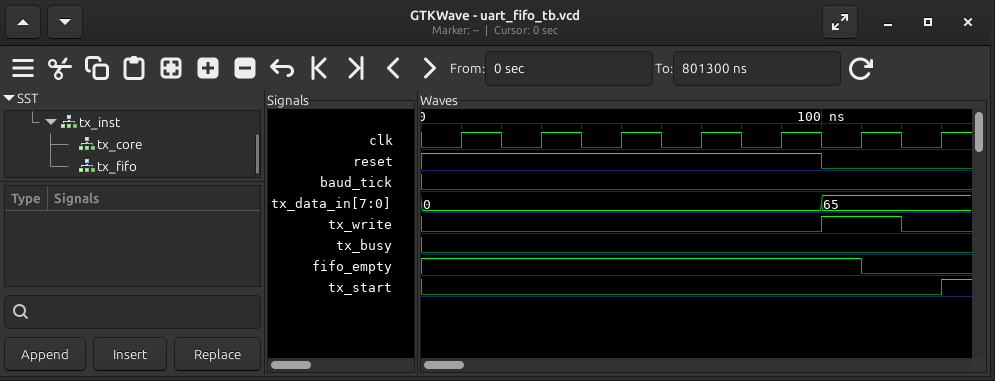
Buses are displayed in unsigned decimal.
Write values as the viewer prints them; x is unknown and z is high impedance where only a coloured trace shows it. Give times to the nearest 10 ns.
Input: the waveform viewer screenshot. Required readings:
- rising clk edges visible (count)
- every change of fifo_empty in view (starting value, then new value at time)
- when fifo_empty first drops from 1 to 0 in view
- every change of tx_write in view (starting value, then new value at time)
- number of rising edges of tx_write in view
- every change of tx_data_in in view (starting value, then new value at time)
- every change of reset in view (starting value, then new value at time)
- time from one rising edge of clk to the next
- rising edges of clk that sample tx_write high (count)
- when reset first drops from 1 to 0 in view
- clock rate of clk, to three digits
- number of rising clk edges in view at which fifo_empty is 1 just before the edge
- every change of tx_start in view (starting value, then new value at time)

7
1, 0 at 110 ns
110 ns
0, 1 at 100 ns, 0 at 120 ns
1
0, 65 at 100 ns
1, 0 at 100 ns
20 ns
1
100 ns
50.0 MHz
6
0, 1 at 130 ns
